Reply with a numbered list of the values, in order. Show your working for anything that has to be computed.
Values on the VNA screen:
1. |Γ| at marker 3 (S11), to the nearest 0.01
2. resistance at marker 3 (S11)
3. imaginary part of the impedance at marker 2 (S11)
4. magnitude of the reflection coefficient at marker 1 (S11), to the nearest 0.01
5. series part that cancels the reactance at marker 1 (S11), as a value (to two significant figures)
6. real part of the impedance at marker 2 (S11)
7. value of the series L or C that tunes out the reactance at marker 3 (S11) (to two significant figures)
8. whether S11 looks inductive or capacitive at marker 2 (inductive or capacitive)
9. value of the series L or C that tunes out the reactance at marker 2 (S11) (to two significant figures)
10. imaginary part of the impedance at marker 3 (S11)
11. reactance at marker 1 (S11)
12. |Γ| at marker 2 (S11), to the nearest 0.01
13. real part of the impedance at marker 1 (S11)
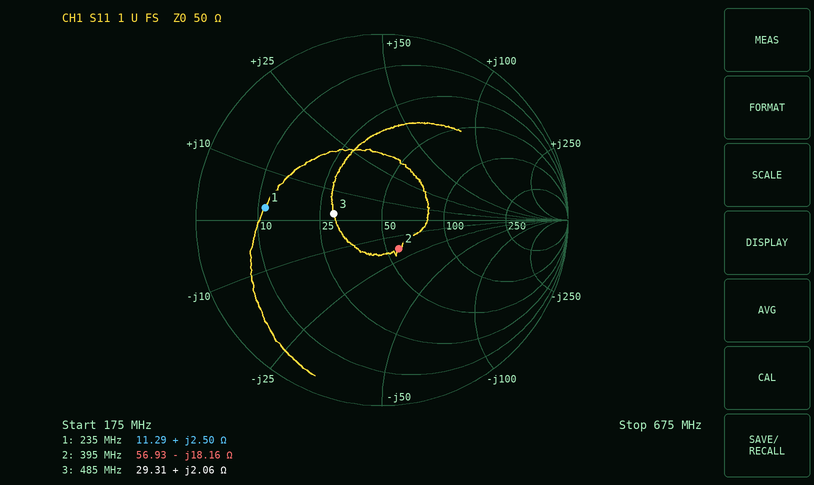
1. 0.26
2. 29.31 Ω
3. -18.16 Ω
4. 0.63
5. C = 1/(2π × 235 MHz × 2.5 Ω) ≈ 271 pF, so 270 pF to two significant figures
6. 56.93 Ω
7. C = 1/(2π × 485 MHz × 2.06 Ω) ≈ 159 pF, so 160 pF to two significant figures
8. capacitive
9. L = 18.16 Ω/(2π × 395 MHz) ≈ 7.3 nH
10. +2.06 Ω
11. +2.50 Ω
12. 0.18
13. 11.29 Ω
